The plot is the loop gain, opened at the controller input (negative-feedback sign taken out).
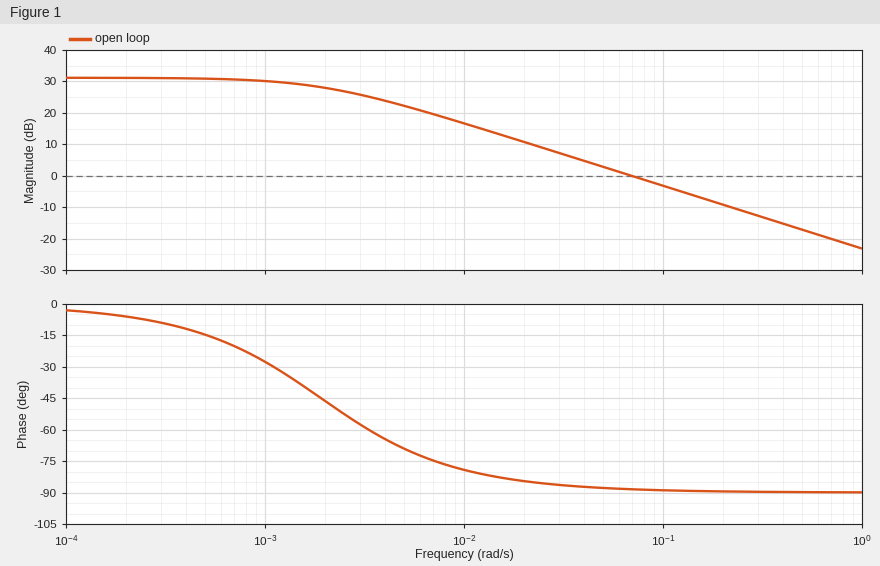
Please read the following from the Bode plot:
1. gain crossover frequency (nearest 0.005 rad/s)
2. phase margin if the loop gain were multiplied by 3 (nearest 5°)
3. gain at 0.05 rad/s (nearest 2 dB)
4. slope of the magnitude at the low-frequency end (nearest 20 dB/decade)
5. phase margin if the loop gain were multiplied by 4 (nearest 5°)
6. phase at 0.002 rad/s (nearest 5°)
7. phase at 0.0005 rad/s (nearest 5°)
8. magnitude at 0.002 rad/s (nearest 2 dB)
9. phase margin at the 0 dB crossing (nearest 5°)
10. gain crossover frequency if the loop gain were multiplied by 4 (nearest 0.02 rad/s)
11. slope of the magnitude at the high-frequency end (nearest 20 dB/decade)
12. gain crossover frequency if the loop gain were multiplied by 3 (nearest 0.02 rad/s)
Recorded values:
0.070 rad/s
90°
2 dB
0 dB/decade
90°
-45°
-15°
28 dB
90°
0.28 rad/s
-20 dB/decade
0.20 rad/s
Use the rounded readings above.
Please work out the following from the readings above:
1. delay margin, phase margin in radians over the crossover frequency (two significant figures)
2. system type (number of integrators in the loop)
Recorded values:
22 s
0
